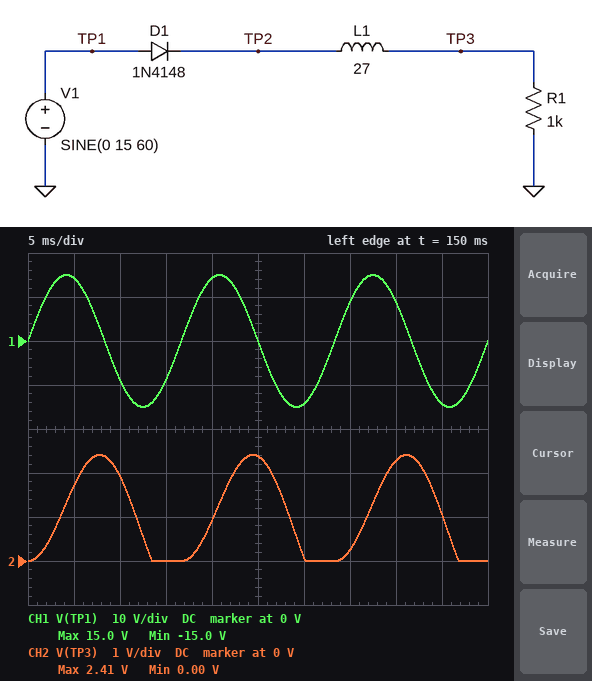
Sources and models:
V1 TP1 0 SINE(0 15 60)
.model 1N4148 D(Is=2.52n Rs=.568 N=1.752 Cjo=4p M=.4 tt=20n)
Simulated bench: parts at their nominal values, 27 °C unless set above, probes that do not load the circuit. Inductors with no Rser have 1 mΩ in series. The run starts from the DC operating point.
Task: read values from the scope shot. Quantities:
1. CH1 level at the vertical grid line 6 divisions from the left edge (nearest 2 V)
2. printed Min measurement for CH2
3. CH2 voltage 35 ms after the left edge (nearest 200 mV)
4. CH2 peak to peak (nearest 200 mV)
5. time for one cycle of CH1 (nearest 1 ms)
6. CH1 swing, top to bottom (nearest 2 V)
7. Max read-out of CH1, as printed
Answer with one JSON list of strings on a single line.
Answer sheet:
["-14 V", "0.00 V", "200 mV", "2.4 V", "17 ms", "30 V", "15.0 V"]
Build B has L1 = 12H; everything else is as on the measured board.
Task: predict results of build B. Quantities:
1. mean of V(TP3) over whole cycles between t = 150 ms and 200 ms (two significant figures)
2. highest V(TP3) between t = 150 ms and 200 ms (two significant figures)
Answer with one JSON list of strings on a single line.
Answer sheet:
["1.9 V", "4.6 V"]
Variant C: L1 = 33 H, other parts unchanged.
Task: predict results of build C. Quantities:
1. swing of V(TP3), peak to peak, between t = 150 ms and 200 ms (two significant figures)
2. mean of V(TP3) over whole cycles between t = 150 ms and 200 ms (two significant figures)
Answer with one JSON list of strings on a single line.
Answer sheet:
["2.0 V", "900 mV"]
